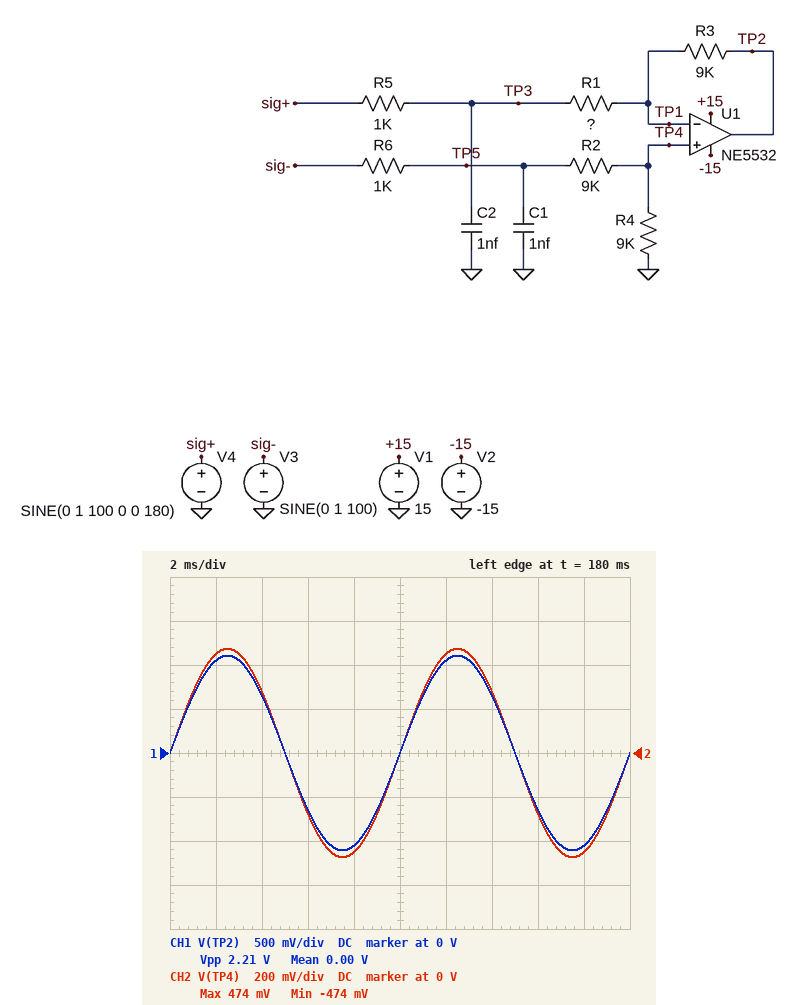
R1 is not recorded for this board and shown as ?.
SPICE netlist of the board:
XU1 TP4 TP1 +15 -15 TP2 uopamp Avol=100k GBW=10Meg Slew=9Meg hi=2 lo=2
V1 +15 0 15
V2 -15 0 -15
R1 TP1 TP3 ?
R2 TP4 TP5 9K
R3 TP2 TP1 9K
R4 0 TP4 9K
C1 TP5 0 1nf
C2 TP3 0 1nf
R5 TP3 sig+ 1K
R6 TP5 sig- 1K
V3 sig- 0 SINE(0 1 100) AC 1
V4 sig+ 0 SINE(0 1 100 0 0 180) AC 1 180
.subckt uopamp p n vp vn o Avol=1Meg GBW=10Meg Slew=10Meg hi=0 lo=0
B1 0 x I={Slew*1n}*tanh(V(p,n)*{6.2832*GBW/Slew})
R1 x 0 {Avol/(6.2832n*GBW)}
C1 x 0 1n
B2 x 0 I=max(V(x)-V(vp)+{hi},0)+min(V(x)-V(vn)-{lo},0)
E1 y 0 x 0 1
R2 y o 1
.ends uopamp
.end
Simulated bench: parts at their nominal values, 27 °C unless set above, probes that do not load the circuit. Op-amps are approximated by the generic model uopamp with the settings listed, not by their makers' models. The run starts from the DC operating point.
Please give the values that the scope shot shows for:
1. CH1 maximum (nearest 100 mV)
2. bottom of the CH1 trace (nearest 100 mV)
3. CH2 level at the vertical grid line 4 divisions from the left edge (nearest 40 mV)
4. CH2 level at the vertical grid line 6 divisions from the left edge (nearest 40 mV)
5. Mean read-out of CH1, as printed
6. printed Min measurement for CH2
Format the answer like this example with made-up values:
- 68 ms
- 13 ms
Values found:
- 1.1 V
- -1.1 V
- -440 mV
- 440 mV
- 0.00 V
- -474 mV
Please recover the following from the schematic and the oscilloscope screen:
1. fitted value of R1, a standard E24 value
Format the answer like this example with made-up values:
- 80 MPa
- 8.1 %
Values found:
- 20 kΩ
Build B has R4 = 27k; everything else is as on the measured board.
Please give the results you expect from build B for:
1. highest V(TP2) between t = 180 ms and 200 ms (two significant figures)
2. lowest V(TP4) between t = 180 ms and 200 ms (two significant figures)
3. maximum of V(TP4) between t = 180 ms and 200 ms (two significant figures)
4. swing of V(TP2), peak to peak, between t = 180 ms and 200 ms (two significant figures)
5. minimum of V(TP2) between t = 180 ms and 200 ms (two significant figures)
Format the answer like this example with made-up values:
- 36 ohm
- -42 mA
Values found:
- 1.5 V
- -730 mV
- 730 mV
- 2.9 V
- -1.5 V
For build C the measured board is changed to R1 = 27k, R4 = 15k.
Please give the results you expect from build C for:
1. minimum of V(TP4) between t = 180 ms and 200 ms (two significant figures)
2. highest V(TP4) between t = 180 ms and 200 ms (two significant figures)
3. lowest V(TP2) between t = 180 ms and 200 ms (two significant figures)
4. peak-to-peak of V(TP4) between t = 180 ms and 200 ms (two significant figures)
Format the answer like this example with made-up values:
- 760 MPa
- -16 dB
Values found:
- -600 mV
- 600 mV
- -1.1 V
- 1.2 V
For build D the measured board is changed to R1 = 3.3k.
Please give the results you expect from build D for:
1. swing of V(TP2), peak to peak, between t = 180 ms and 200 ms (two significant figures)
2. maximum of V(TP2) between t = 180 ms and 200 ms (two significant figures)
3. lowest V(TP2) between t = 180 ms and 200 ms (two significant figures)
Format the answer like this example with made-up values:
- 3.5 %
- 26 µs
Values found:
- 7.1 V
- 3.6 V
- -3.6 V
